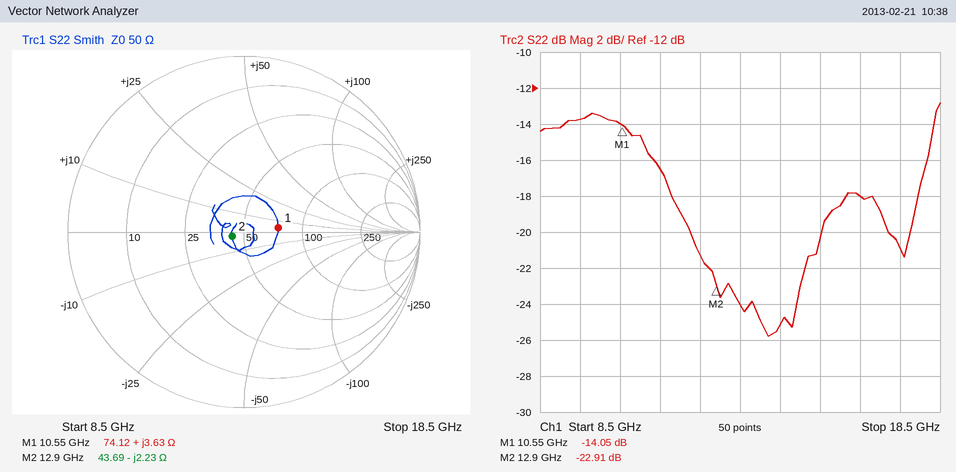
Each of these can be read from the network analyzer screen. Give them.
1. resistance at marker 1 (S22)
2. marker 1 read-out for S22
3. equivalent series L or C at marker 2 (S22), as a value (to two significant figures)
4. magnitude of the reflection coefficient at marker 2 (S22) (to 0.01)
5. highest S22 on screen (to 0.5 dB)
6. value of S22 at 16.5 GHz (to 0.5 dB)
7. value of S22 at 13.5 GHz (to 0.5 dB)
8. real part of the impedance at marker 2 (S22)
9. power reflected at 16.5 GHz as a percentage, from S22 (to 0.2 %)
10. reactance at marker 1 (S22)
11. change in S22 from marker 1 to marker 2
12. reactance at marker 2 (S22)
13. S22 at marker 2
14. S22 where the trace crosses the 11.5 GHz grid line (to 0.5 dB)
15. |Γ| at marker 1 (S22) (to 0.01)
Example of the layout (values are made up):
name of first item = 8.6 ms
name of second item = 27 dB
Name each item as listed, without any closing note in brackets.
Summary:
resistance at marker 1 = 74.12 Ω
marker 1 read-out for S22 = -14.05 dB
equivalent series L or C at marker 2 (S22), as a value = 5.5 pF
magnitude of the reflection coefficient at marker 2 (S22) = 0.07
highest S22 on screen = -13.0 dB
value of S22 at 16.5 GHz = -18.0 dB
value of S22 at 13.5 GHz = -24.0 dB
real part of the impedance at marker 2 = 43.69 Ω
power reflected at 16.5 GHz as a percentage, from S22 = 1.6 %
reactance at marker 1 = +3.63 Ω
change in S22 from marker 1 to marker 2 = -8.86 dB
reactance at marker 2 = -2.23 Ω
S22 at marker 2 = -22.91 dB
S22 where the trace crosses the 11.5 GHz grid line = -16.5 dB
|Γ| at marker 1 (S22) = 0.20
